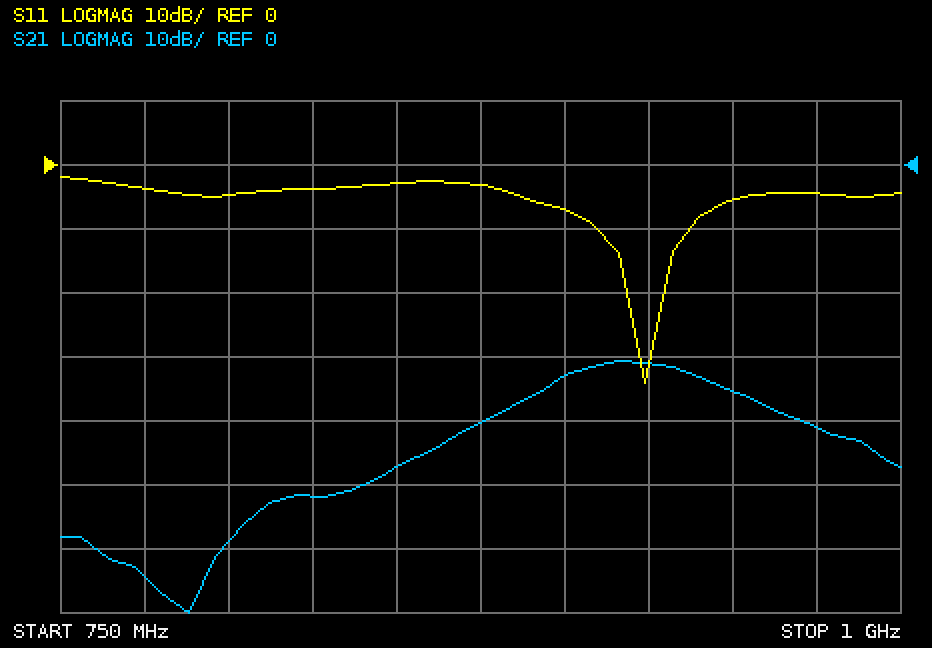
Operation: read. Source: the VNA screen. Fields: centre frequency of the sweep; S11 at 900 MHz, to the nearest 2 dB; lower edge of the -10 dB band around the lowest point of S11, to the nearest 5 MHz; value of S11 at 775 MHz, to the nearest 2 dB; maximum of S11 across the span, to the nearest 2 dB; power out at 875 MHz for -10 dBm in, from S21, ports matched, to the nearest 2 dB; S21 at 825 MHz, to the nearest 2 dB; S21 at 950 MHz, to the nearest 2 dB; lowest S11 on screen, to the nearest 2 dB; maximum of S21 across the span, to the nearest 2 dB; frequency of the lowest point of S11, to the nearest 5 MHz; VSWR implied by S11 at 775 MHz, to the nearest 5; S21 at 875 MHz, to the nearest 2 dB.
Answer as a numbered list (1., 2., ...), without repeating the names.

1. 875 MHz
2. -6 dB
3. 910 MHz
4. -4 dB
5. -2 dB
6. -50 dBm
7. -52 dB
8. -36 dB
9. -34 dB
10. -30 dB
11. 925 MHz
12. 5
13. -40 dB
